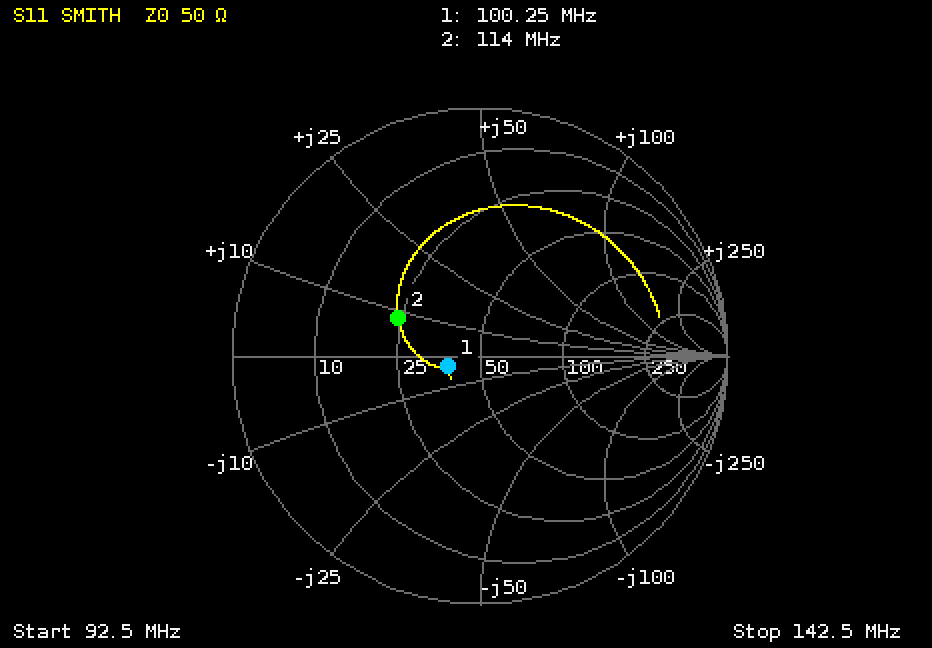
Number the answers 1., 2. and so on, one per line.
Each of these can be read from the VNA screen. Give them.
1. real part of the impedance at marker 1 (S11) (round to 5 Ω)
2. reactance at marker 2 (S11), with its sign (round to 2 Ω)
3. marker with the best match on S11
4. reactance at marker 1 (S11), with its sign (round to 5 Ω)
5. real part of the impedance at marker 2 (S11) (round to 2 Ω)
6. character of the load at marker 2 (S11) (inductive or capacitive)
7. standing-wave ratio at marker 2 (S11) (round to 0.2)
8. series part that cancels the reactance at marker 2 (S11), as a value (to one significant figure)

1. 40 Ω
2. +8 Ω
3. marker 1
4. -5 Ω
5. 24 Ω
6. inductive
7. 2.2
8. 200 pF
